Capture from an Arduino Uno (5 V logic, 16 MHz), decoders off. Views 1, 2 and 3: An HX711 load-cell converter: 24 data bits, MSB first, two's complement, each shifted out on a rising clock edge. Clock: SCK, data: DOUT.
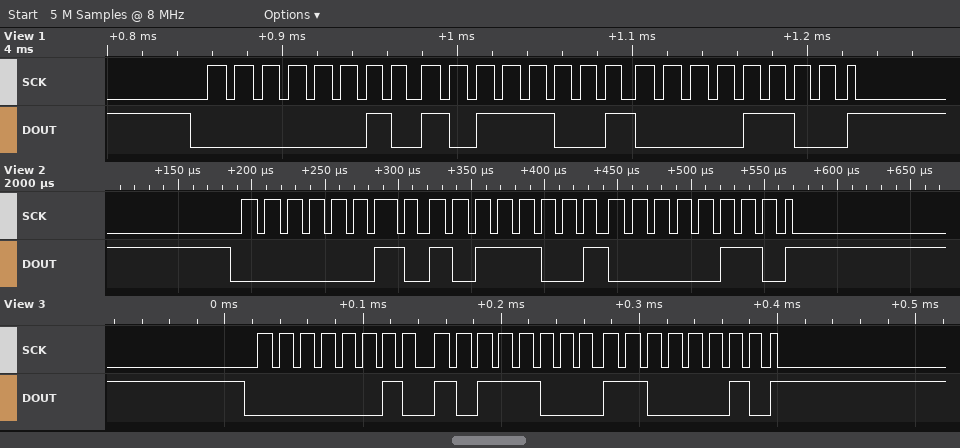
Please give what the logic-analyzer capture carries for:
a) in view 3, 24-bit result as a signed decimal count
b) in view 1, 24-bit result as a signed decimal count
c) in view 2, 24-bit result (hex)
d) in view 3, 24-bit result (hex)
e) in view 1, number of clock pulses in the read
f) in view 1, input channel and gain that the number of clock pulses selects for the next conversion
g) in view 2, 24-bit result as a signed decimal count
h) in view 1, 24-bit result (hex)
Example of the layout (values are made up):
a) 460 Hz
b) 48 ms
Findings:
a) 178370
b) 178444
c) 0x02B906
d) 0x02B8C2
e) 25
f) channel A, gain 128
g) 178438
h) 0x02B90C
